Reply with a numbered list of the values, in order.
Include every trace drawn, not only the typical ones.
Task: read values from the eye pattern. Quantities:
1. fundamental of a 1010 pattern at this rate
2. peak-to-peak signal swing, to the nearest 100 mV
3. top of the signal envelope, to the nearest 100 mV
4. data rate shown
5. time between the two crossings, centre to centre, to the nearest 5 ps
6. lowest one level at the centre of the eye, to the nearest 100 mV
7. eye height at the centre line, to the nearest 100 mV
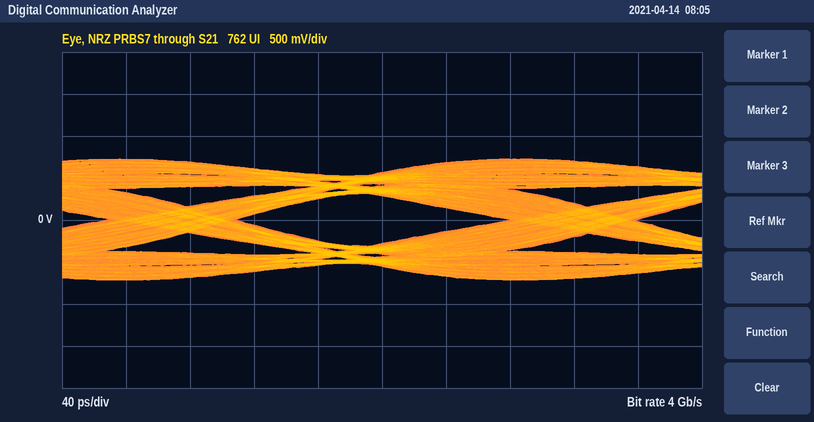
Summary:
1. 2 GHz
2. 1.4 V
3. 700 mV
4. 4 Gb/s
5. 250 ps
6. 300 mV
7. 600 mV
